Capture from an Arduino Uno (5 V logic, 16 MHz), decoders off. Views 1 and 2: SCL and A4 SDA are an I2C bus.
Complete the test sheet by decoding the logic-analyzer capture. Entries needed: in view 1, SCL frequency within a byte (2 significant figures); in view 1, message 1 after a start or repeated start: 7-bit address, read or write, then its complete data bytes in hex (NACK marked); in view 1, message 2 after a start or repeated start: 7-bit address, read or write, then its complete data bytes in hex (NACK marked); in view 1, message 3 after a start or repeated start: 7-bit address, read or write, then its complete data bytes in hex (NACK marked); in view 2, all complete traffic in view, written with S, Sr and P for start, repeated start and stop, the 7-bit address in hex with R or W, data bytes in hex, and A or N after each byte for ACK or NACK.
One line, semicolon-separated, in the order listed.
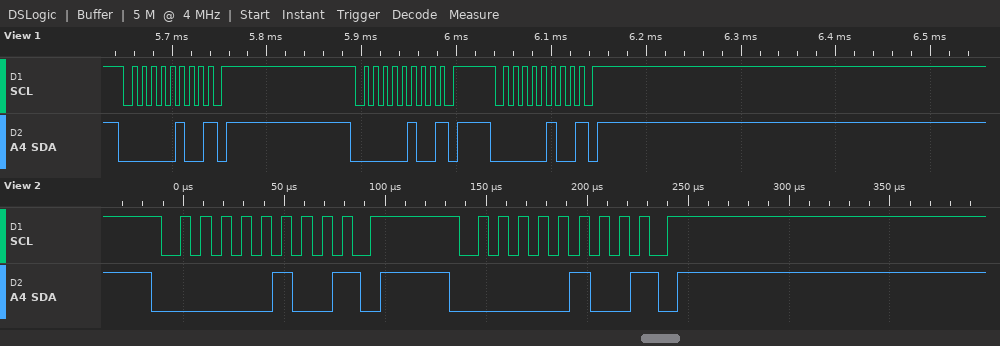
100 kHz; 0x02 write NACK; 0x02 write NACK; 0x02 write NACK; S 02W N P S 02W N P
